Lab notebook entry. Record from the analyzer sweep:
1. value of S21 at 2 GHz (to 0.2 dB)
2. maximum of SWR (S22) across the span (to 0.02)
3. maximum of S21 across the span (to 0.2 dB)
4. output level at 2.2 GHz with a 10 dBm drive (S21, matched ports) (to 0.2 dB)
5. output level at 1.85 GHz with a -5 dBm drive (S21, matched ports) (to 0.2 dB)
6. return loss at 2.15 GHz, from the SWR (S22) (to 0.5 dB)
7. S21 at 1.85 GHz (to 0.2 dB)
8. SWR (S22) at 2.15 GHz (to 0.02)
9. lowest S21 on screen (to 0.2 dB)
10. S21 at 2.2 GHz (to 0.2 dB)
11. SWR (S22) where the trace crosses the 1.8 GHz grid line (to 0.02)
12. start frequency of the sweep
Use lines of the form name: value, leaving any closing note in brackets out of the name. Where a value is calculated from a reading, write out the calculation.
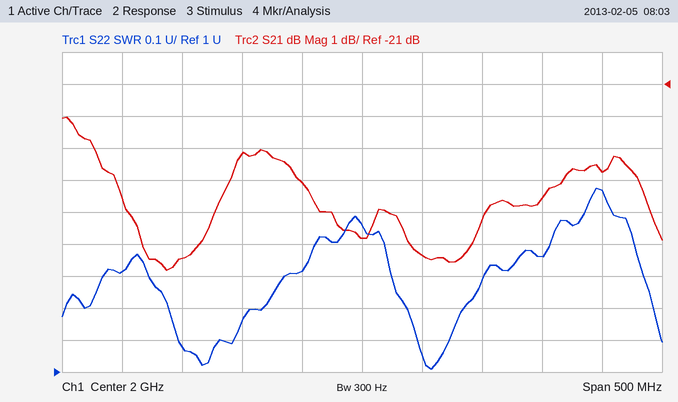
value of S21 at 2 GHz: -25.8 dB
maximum of SWR (S22) across the span: 1.58
maximum of S21 across the span: -22.0 dB
output level at 2.2 GHz with a 10 dBm drive (S21, matched ports): 10 dBm + (-23.8 dB) = -13.8 dBm
output level at 1.85 GHz with a -5 dBm drive (S21, matched ports): -5 dBm + (-26.4 dB) = -31.4 dBm
return loss at 2.15 GHz, from the SWR (S22): −20 log10((1.36 − 1)/(1.36 + 1)) ≈ 16.3 dB, so 16.5 dB to the nearest 0.5 dB
S21 at 1.85 GHz: -26.4 dB
SWR (S22) at 2.15 GHz: 1.36
lowest S21 on screen: -26.8 dB
S21 at 2.2 GHz: -23.8 dB
SWR (S22) where the trace crosses the 1.8 GHz grid line: 1.32
start frequency of the sweep: 1.75 GHz
